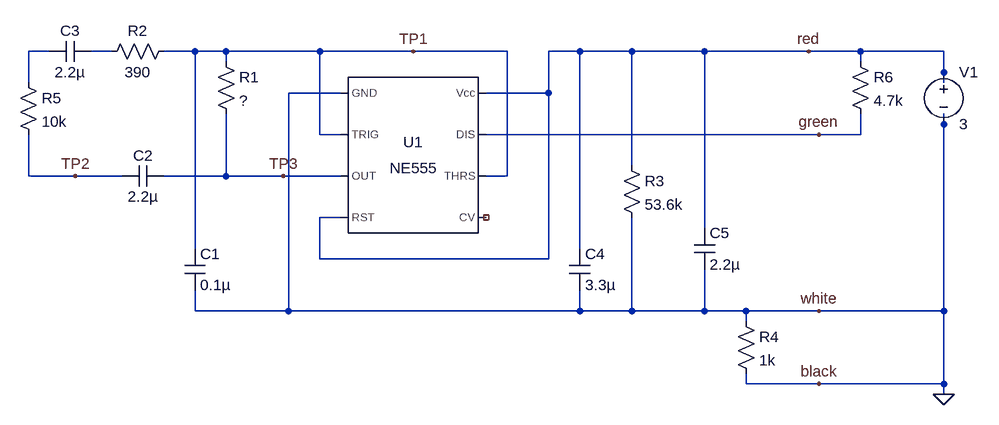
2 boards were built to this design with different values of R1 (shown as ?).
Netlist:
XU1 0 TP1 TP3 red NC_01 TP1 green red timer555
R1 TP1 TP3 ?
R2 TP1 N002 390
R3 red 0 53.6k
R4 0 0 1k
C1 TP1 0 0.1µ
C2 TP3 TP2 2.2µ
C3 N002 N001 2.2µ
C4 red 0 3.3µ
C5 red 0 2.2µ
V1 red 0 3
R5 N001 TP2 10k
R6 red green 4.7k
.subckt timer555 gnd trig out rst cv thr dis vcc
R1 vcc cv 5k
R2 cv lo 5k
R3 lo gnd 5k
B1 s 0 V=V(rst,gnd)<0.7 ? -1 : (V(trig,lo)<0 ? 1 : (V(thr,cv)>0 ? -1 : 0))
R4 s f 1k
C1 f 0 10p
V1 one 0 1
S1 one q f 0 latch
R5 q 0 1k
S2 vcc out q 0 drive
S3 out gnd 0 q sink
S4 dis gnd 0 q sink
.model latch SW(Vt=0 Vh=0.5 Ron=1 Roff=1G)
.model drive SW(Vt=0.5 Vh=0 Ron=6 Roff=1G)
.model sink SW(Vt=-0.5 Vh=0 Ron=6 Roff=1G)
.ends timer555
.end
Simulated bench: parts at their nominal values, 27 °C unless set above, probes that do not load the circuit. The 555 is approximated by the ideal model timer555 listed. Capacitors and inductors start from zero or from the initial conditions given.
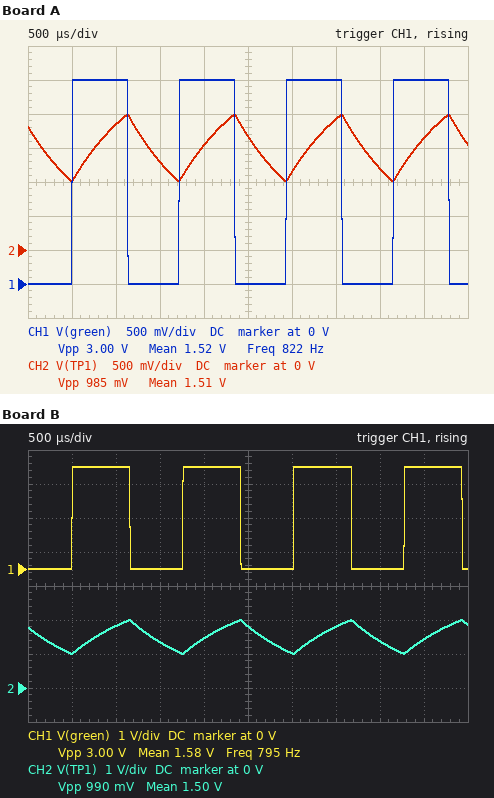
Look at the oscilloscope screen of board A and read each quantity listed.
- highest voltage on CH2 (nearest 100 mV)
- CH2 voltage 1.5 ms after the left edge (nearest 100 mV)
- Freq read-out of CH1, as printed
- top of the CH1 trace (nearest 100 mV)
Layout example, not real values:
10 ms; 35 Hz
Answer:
2.0 V; 1.3 V; 822 Hz; 3.0 V
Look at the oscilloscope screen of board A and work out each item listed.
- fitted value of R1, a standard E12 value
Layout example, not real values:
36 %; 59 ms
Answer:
56 kΩ
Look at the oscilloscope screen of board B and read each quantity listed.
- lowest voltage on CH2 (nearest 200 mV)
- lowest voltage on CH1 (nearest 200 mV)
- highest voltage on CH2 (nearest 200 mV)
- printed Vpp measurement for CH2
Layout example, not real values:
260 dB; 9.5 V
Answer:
1.0 V; 0 V; 2.0 V; 990 mV
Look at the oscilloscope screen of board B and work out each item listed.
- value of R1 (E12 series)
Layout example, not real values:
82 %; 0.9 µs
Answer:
68 kΩ
